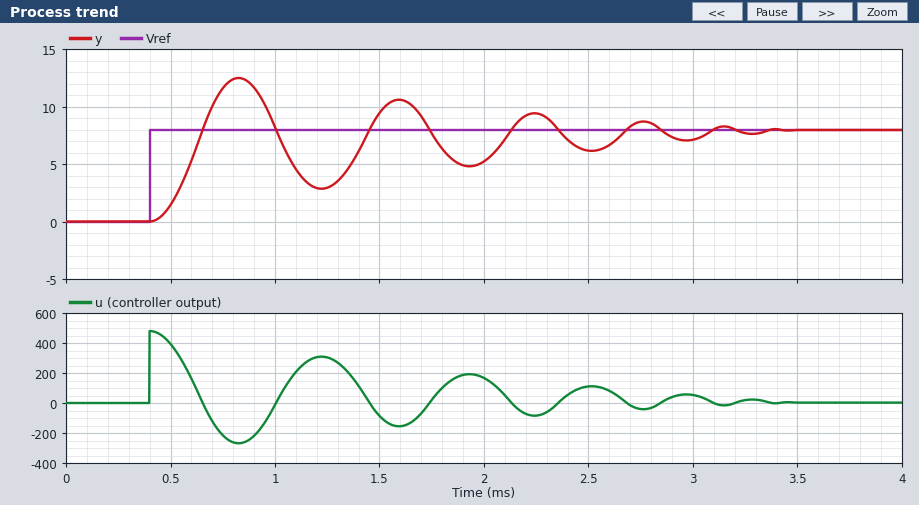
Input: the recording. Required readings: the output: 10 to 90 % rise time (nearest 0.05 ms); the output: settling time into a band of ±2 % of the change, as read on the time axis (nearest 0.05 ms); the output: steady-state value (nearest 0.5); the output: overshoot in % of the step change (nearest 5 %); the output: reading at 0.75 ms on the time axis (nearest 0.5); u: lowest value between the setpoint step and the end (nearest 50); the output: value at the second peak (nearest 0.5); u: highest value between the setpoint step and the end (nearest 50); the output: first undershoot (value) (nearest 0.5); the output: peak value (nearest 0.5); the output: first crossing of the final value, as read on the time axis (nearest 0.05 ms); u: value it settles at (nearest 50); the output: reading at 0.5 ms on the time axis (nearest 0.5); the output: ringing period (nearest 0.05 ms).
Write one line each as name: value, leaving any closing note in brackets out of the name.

the output: 10 to 90 % rise time: 0.15 ms
the output: settling time into a band of ±2 % of the change, as read on the time axis: 3.35 ms
the output: steady-state value: 8.0
the output: overshoot in % of the step change: 55 %
the output: reading at 0.75 ms on the time axis: 11.5
u: lowest value between the setpoint step and the end: -250
the output: value at the second peak: 10.5
u: highest value between the setpoint step and the end: 500
the output: first undershoot (value): 3.0
the output: peak value: 12.5
the output: first crossing of the final value, as read on the time axis: 0.65 ms
u: value it settles at: 0
the output: reading at 0.5 ms on the time axis: 1.5
the output: ringing period: 0.75 ms
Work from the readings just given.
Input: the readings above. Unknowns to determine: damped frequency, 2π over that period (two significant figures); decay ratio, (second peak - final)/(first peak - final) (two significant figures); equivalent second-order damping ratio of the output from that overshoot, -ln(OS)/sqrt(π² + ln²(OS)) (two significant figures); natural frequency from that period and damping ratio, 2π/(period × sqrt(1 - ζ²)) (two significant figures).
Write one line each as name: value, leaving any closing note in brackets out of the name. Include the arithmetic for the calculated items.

damped frequency, 2π over that period: 2π / 0.75 = 8.4 rad/ms
decay ratio, (second peak - final)/(first peak - final): (10.5 - 8) / (12.5 - 8) = 0.56
equivalent second-order damping ratio of the output from that overshoot, -ln(OS)/sqrt(π² + ln²(OS)): ln(0.55) = -0.598; 0.598 / sqrt(9.870 + 0.357) = 0.19
natural frequency from that period and damping ratio, 2π/(period × sqrt(1 - ζ²)): 2π / (0.75 × sqrt(1 - 0.19²)) = 8.5 rad/ms
